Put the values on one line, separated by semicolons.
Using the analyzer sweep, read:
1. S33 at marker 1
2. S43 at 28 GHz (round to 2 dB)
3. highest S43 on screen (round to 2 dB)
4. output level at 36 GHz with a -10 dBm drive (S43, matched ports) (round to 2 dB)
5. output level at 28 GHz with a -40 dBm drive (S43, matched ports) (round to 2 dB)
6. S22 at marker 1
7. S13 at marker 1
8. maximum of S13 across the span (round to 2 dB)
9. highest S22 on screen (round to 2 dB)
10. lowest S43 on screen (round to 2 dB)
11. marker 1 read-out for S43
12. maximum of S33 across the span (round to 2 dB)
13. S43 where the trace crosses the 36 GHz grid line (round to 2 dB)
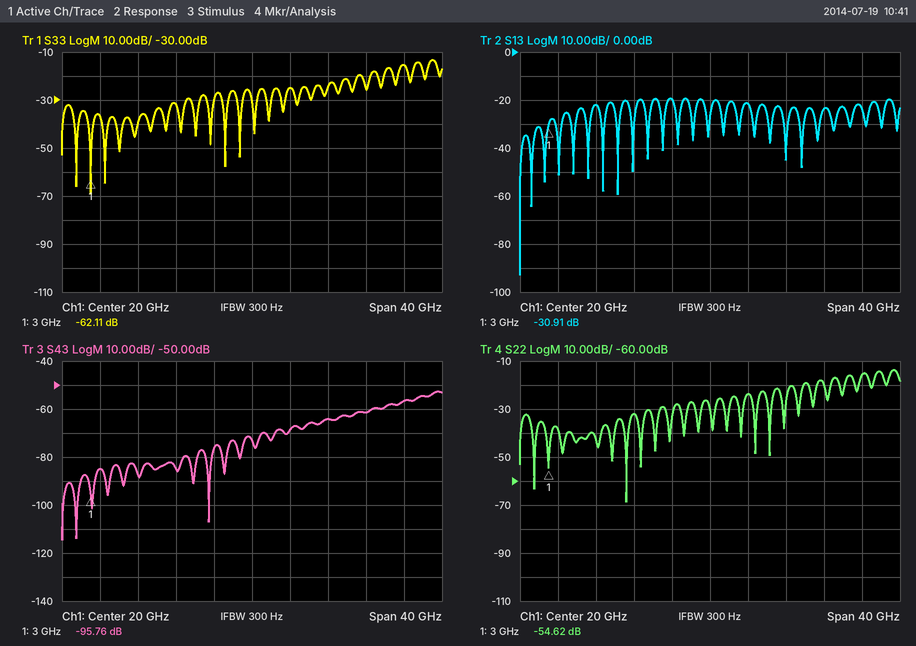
-62.11 dB; -64 dB; -52 dB; -66 dBm; -104 dBm; -54.62 dB; -30.91 dB; -20 dB; -14 dB; -114 dB; -95.76 dB; -14 dB; -56 dB
